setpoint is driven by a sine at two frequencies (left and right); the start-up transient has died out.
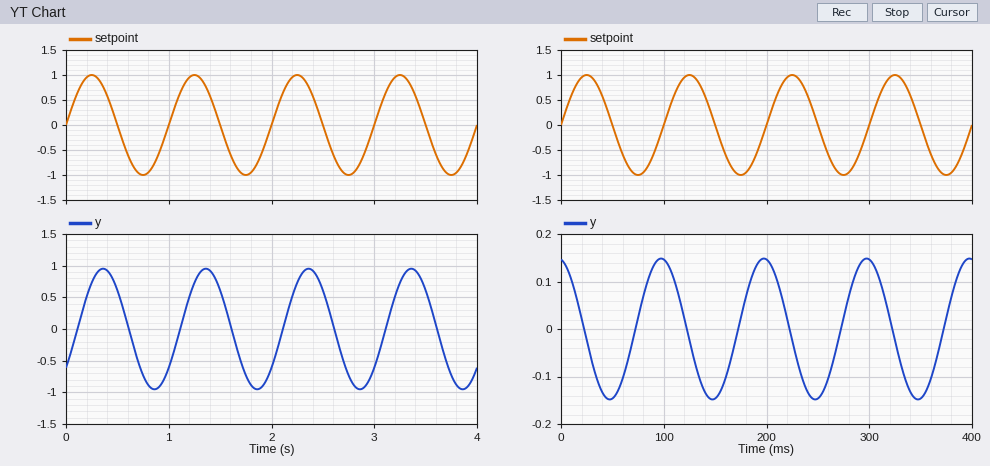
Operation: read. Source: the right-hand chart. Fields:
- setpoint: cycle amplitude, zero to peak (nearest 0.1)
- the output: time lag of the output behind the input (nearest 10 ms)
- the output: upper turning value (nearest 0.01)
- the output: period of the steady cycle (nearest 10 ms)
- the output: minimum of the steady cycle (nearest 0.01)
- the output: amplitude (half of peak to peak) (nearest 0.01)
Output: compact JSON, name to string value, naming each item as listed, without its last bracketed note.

{"setpoint: cycle amplitude, zero to peak": "1.0", "the output: time lag of the output behind the input": "70 ms", "the output: upper turning value": "0.15", "the output: period of the steady cycle": "100 ms", "the output: minimum of the steady cycle": "-0.15", "the output: amplitude (half of peak to peak)": "0.15"}
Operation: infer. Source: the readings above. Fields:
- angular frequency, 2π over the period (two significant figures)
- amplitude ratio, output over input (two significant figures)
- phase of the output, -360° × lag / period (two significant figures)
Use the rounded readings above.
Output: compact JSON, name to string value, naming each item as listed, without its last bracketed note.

{"angular frequency, 2π over the period": "0.063 rad/ms", "amplitude ratio, output over input": "0.15", "phase of the output, -360° × lag / period": "-250°"}
